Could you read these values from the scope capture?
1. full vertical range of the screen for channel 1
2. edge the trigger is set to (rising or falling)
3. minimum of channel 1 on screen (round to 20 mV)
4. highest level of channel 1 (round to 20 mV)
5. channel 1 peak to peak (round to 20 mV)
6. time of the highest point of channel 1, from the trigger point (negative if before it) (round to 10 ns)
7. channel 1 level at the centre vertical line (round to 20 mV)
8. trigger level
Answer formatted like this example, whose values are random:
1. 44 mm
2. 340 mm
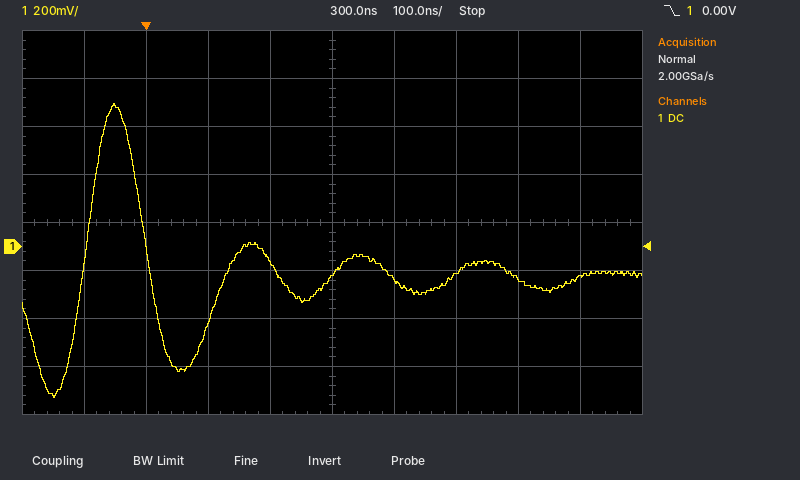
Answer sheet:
1. 1.6 V
2. falling
3. -620 mV
4. 600 mV
5. 1.22 V
6. -50 ns
7. -120 mV
8. 0.00 V
